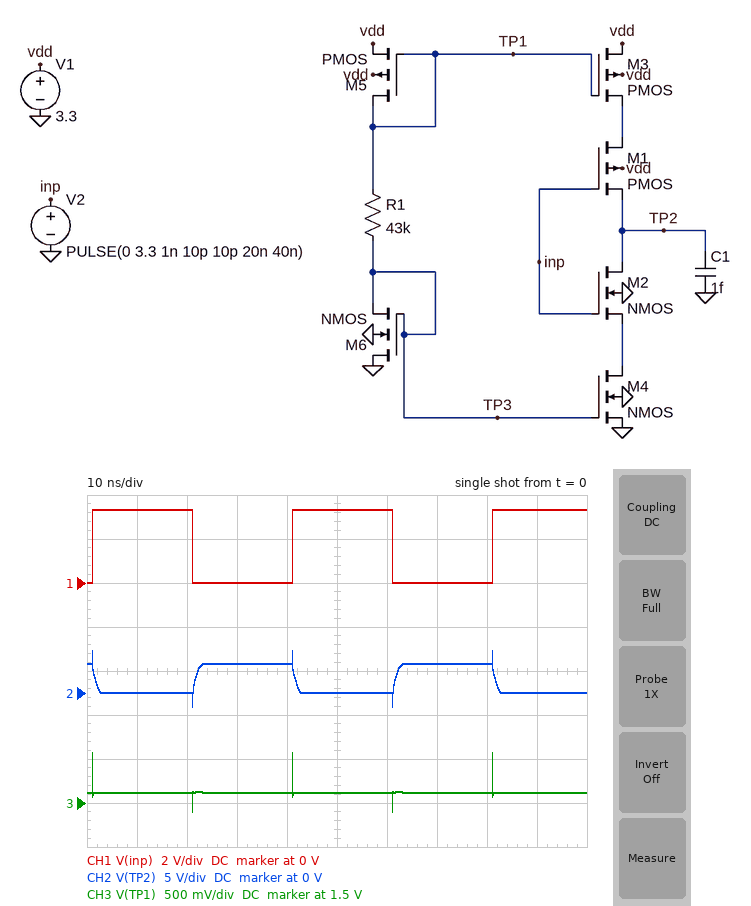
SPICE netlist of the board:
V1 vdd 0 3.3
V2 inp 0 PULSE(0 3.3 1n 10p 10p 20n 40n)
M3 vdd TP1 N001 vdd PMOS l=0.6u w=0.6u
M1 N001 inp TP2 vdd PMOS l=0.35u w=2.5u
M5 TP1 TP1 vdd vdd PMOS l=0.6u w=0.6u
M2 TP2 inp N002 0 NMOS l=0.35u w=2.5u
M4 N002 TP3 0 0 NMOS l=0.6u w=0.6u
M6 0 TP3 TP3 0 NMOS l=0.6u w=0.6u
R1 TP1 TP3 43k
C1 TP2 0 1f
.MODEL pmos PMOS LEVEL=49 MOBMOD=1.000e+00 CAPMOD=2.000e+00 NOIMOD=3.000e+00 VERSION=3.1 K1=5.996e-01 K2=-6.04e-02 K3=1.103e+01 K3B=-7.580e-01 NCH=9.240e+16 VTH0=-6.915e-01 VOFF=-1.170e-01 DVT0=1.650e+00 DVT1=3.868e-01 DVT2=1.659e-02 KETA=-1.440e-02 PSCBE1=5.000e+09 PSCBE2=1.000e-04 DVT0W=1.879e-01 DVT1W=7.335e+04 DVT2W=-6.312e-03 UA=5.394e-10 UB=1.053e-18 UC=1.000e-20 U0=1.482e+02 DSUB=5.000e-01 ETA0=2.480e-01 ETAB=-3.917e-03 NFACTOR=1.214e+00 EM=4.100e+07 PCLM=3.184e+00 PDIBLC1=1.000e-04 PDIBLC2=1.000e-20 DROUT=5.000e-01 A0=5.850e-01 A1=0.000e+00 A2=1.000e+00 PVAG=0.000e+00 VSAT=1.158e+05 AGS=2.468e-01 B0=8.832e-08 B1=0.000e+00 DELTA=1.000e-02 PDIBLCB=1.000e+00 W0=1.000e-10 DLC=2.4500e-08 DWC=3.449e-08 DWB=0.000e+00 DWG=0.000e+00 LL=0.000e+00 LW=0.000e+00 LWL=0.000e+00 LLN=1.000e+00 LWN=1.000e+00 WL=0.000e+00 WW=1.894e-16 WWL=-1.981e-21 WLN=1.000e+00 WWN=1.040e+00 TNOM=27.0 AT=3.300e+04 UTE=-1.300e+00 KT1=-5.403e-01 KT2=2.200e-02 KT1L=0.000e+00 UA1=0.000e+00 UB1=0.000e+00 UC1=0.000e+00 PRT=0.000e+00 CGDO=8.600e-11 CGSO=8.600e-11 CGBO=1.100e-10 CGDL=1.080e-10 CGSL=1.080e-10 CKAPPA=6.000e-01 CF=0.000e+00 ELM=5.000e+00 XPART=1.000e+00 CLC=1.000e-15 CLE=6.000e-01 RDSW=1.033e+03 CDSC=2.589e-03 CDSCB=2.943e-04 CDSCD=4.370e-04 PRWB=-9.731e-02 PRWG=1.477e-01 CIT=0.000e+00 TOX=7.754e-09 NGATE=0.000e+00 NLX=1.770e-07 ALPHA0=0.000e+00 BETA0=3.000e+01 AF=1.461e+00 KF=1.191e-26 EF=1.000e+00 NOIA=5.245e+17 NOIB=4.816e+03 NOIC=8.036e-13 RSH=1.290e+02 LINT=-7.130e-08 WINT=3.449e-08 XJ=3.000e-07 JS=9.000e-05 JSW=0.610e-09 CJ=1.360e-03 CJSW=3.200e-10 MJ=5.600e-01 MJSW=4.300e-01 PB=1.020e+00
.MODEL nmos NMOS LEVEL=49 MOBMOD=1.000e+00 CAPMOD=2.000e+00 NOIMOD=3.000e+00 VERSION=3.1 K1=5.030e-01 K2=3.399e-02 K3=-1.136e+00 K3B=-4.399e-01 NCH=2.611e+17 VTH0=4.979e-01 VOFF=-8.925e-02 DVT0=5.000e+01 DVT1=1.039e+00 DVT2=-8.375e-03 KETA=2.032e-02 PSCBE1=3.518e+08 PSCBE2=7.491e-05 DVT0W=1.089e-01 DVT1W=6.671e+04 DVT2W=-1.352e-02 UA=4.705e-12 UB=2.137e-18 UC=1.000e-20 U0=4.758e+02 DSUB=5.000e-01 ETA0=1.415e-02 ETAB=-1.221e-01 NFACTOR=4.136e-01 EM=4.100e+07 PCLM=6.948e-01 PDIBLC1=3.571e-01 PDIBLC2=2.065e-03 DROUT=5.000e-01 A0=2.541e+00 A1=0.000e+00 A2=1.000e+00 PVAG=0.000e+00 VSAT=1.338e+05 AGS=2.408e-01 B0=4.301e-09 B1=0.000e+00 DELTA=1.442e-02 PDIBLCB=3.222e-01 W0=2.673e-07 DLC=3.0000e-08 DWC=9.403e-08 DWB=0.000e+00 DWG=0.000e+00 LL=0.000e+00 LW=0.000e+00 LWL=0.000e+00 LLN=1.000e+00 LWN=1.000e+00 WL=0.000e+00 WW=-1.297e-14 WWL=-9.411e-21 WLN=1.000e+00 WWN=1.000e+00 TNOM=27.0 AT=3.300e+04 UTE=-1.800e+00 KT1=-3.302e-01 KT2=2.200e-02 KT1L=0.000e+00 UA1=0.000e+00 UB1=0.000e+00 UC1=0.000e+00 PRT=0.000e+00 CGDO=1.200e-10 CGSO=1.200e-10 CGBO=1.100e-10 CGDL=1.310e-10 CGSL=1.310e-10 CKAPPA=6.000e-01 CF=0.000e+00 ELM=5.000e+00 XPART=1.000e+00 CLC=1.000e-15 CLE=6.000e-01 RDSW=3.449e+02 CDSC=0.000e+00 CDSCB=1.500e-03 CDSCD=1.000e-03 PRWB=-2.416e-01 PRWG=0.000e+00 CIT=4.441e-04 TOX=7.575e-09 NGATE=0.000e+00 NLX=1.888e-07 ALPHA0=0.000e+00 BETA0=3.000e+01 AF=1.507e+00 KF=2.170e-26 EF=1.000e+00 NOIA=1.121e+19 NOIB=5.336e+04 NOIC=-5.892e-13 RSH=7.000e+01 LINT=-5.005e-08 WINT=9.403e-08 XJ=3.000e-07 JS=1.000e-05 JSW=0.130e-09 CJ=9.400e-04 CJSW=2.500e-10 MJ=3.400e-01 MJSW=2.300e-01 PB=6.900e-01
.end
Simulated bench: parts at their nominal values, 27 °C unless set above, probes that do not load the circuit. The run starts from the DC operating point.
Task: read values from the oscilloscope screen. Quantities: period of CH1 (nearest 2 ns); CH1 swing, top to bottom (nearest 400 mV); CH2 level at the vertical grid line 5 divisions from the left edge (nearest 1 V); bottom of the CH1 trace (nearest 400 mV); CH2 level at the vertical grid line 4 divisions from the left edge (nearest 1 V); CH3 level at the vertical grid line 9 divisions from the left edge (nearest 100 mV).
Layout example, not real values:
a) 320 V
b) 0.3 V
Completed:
a) 40 ns
b) 3.2 V
c) 0 V
d) 0 V
e) 3 V
f) 1.6 V
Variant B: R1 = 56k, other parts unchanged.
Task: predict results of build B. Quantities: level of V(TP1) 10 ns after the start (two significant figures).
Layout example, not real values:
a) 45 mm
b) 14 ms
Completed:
a) 1.7 V
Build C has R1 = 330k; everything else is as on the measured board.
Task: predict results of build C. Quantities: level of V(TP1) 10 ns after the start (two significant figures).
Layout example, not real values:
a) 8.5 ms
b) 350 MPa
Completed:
a) 2.1 V
